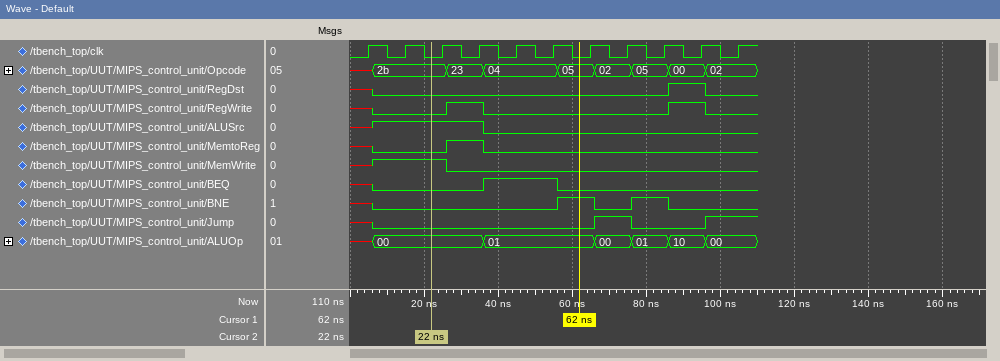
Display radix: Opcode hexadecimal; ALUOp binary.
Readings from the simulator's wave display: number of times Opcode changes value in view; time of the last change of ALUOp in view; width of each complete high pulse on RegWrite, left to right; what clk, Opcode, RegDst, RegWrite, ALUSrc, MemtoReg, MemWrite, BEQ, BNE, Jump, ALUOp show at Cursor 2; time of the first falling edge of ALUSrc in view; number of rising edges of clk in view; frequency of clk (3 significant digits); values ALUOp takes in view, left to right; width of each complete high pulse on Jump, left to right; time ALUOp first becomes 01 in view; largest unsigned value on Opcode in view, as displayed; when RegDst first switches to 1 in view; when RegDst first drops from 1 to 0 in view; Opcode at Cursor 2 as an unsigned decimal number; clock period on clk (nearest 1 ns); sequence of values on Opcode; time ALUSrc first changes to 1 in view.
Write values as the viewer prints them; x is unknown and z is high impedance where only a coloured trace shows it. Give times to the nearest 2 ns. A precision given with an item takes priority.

8
96 ns
10 ns, 10 ns
clk=0, Opcode=2b, RegDst=0, RegWrite=0, ALUSrc=1, MemtoReg=0, MemWrite=1, BEQ=0, BNE=0, Jump=0, ALUOp=00
36 ns
11
100 MHz
x, 00, 01, 00, 01, 10, 00
10 ns
36 ns
2b
86 ns
96 ns
43
10 ns
x, 2b, 23, 04, 05, 02, 05, 00, 02
6 ns
